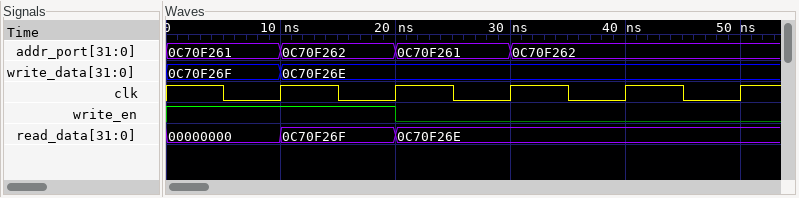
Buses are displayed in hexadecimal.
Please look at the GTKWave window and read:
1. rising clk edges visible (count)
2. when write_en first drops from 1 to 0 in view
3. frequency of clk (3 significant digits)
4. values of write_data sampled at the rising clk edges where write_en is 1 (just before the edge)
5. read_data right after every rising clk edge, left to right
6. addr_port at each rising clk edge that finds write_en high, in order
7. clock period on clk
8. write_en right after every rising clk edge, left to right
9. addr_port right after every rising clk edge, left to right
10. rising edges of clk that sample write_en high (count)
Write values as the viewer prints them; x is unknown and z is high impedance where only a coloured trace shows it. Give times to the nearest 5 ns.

5
20 ns
100 MHz
0C70F26F, 0C70F26E
0C70F26F, 0C70F26E, 0C70F26E, 0C70F26E, 0C70F26E
0C70F261, 0C70F262
10 ns
1 0 0 0 0
0C70F262, 0C70F261, 0C70F262, 0C70F262, 0C70F262
2
